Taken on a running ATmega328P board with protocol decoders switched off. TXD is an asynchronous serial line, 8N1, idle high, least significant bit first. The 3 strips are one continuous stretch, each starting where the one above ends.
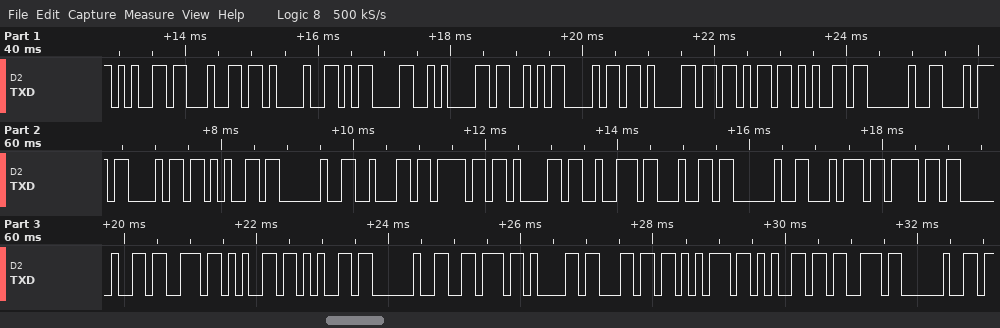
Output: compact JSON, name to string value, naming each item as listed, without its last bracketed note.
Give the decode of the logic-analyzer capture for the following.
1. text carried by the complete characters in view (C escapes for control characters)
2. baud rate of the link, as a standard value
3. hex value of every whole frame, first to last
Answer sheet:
{"text carried by the complete characters in view": "\"ed!\\r\\nShake the board to see values \"", "baud rate of the link, as a standard value": "9600 baud", "hex value of every whole frame, first to last": "0x65 0x64 0x21 0x0D 0x0A 0x53 0x68 0x61 0x6B 0x65 0x20 0x74 0x68 0x65 0x20 0x62 0x6F 0x61 0x72 0x64 0x20 0x74 0x6F 0x20 0x73 0x65 0x65 0x20 0x76 0x61 0x6C 0x75 0x65 0x73 0x20"}
